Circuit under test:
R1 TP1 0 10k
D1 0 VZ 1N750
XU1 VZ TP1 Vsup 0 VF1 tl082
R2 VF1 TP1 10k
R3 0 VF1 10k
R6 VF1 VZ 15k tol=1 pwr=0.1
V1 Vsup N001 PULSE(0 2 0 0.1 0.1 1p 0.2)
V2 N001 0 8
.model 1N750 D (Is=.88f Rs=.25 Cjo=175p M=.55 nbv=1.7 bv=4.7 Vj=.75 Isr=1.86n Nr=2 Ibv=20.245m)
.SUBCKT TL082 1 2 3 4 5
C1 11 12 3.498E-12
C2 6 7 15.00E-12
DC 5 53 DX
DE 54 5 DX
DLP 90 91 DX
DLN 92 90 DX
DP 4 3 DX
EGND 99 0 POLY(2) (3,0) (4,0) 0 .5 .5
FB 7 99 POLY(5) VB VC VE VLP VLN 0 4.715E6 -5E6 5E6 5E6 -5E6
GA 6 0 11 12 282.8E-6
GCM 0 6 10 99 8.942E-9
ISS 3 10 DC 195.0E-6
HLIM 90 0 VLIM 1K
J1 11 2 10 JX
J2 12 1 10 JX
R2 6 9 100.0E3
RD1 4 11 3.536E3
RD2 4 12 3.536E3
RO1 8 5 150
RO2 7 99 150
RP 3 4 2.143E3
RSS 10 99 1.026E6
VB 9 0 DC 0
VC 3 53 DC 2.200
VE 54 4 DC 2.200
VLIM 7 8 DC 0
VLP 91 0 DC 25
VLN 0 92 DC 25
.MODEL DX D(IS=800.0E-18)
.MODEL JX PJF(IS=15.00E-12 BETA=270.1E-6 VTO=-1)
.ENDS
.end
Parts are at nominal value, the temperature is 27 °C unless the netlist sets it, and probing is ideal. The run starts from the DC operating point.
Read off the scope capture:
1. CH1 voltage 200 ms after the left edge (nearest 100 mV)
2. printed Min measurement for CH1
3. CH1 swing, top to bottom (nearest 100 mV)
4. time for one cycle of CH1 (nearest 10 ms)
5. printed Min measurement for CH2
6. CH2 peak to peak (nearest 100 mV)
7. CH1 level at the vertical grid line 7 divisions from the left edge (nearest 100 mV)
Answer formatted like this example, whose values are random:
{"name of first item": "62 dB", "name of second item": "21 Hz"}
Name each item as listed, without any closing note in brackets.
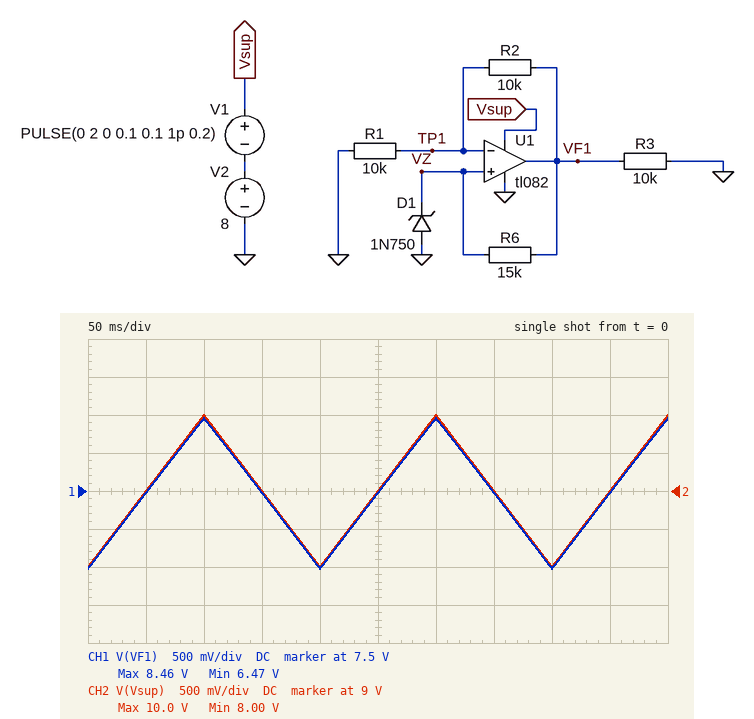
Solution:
{"CH1 voltage 200 ms after the left edge": "6.5 V", "printed Min measurement for CH1": "6.47 V", "CH1 swing, top to bottom": "2.0 V", "time for one cycle of CH1": "200 ms", "printed Min measurement for CH2": "8.00 V", "CH2 peak to peak": "2.0 V", "CH1 level at the vertical grid line 7 divisions from the left edge": "7.5 V"}
